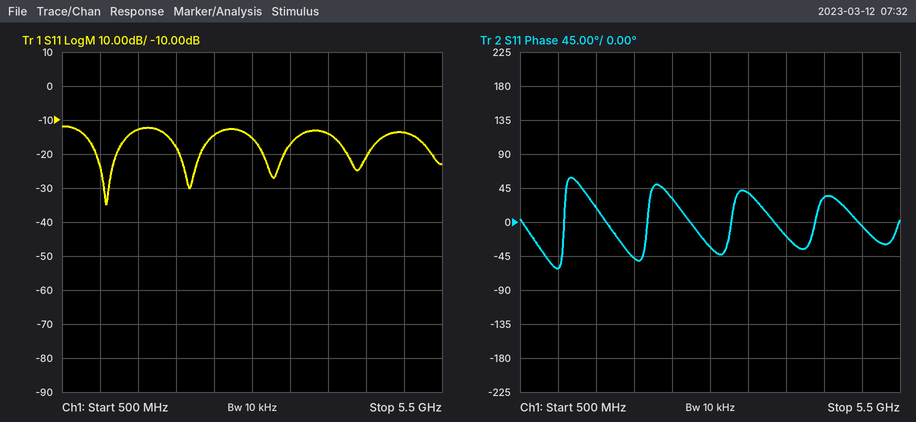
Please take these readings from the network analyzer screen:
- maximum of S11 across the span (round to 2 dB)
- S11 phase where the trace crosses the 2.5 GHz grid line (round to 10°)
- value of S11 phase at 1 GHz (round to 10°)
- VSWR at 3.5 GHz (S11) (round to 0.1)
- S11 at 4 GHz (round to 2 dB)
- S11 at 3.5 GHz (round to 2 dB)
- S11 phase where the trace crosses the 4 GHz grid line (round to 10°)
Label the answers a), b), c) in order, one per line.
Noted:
a) -12 dB
b) 30°
c) -60°
d) 1.3
e) -14 dB
f) -18 dB
g) -20°
